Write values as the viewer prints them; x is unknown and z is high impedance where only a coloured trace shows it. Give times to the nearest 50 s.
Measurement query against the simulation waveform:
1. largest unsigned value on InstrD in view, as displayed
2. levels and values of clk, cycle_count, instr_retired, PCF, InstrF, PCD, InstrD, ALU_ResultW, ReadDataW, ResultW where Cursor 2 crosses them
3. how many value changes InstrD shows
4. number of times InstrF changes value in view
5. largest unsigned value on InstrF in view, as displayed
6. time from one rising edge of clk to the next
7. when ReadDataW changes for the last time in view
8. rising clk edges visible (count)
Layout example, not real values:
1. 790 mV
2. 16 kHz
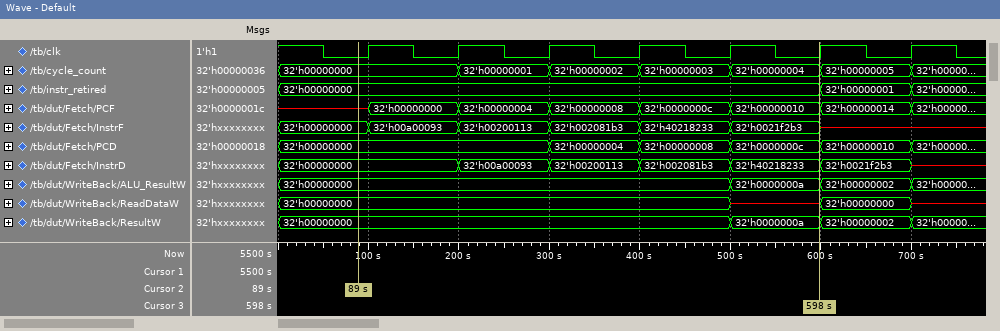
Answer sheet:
1. 32'h40218233
2. clk=0, cycle_count=32'h00000000, instr_retired=32'h00000000, PCF=x, InstrF=32'h00000000, PCD=32'h00000000, InstrD=32'h00000000, ALU_ResultW=32'h00000000, ReadDataW=32'h00000000, ResultW=32'h00000000
3. 6
4. 6
5. 32'h40218233
6. 100 s
7. 700 s
8. 7
